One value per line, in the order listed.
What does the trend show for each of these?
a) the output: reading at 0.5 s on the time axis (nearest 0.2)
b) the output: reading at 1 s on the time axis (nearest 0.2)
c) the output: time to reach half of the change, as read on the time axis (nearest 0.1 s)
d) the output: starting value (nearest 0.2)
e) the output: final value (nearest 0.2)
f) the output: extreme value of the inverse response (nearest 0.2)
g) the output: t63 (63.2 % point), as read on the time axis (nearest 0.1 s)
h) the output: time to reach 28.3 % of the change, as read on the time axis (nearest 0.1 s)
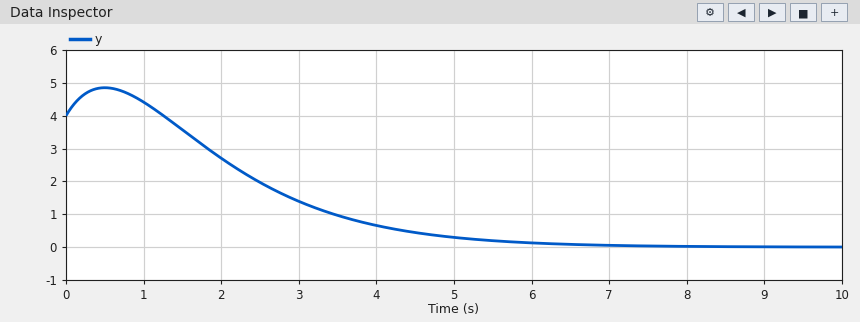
4.8
4.4
2.5 s
4.0
0.0
4.8
2.9 s
1.9 s
